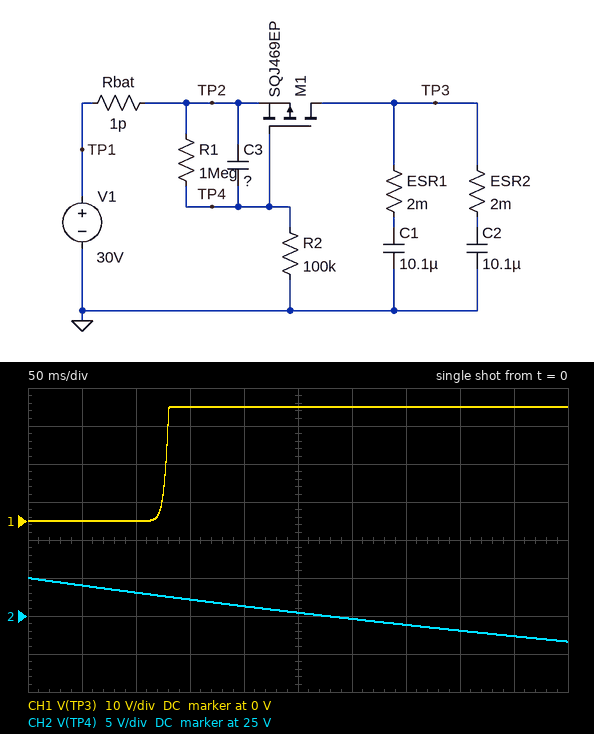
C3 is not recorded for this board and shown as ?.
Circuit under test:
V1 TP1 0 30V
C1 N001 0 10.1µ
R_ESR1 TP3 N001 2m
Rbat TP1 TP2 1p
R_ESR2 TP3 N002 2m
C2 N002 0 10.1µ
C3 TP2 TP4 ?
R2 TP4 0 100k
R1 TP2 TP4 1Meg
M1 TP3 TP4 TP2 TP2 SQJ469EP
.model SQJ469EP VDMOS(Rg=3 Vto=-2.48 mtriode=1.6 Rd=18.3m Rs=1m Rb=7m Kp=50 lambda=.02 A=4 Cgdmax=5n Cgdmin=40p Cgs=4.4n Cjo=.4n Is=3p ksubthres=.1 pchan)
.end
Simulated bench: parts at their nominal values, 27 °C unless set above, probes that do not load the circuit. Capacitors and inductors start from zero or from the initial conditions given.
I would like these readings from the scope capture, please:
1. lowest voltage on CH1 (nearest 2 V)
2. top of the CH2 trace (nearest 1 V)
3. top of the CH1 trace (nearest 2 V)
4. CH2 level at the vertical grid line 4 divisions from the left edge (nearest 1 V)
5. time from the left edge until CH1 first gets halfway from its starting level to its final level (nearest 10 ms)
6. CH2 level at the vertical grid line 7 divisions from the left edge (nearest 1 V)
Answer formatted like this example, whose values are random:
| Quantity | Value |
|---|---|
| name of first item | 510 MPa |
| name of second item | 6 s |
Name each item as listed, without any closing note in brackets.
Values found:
| Quantity | Value |
|---|---|
| lowest voltage on CH1 | 0 V |
| top of the CH2 trace | 30 V |
| top of the CH1 trace | 30 V |
| CH2 level at the vertical grid line 4 divisions from the left edge | 26 V |
| time from the left edge until CH1 first gets halfway from its starting level to its final level | 130 ms |
| CH2 level at the vertical grid line 7 divisions from the left edge | 24 V |
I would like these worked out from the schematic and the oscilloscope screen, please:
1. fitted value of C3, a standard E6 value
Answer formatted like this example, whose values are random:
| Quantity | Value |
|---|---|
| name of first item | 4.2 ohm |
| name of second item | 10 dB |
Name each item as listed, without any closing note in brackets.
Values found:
| Quantity | Value |
|---|---|
| fitted value of C3, a standard E6 value | 15 µF |
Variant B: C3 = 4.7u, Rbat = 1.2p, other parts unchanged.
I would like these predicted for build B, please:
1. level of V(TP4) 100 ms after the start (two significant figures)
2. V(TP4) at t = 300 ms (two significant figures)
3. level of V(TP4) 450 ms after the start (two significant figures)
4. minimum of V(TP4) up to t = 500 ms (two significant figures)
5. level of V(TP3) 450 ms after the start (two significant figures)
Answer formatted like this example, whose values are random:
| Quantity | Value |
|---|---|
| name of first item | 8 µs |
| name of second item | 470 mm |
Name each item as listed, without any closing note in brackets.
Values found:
| Quantity | Value |
|---|---|
| level of V(TP4) 100 ms after the start | 24 V |
| V(TP4) at t = 300 ms | 16 V |
| level of V(TP4) 450 ms after the start | 12 V |
| minimum of V(TP4) up to t = 500 ms | 11 V |
| level of V(TP3) 450 ms after the start | 30 V |
